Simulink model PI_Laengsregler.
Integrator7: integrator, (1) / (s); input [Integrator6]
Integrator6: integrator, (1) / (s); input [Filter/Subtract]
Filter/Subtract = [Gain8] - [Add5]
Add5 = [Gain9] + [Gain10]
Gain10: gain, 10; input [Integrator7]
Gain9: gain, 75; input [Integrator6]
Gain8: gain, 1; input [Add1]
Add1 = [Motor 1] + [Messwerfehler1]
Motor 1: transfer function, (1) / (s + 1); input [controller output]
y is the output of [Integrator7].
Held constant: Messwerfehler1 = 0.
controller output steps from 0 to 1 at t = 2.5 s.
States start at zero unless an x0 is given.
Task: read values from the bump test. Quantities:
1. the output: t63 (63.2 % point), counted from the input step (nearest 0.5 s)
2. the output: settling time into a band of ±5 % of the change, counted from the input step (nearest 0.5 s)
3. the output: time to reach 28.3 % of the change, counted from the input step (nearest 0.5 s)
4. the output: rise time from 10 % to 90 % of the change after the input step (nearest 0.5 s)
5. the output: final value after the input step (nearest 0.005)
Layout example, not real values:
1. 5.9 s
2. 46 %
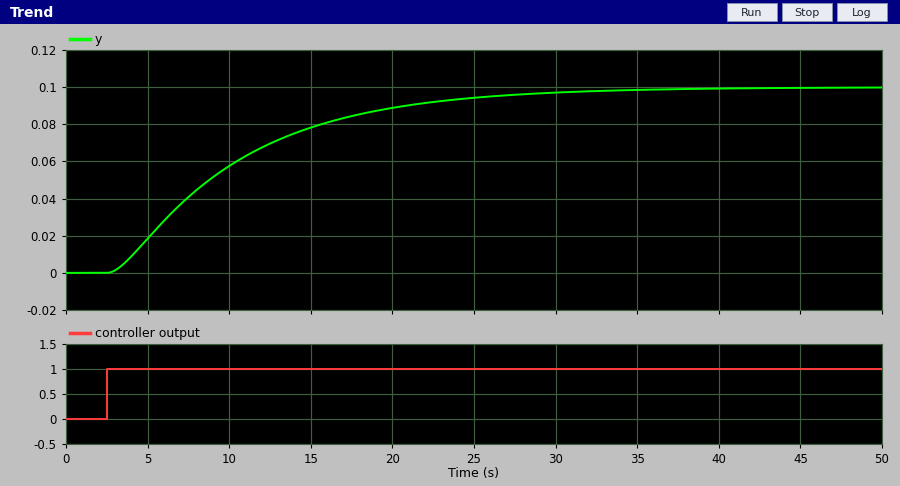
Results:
1. 8.5 s
2. 23.5 s
3. 3.5 s
4. 16.5 s
5. 0.100
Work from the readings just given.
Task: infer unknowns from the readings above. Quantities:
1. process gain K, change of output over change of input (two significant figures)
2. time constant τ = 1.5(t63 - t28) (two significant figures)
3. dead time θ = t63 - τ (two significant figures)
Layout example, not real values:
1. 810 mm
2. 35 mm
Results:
1. 0.10
2. 7.5 s
3. 1.0 s
